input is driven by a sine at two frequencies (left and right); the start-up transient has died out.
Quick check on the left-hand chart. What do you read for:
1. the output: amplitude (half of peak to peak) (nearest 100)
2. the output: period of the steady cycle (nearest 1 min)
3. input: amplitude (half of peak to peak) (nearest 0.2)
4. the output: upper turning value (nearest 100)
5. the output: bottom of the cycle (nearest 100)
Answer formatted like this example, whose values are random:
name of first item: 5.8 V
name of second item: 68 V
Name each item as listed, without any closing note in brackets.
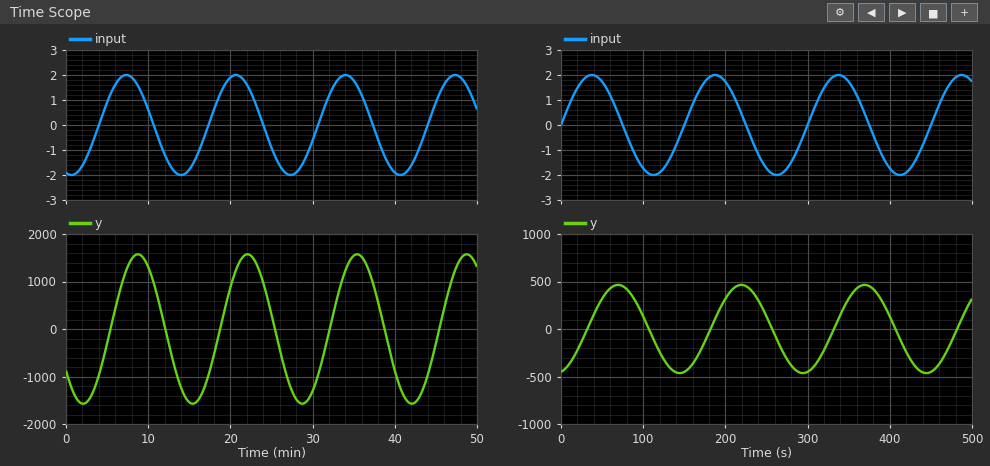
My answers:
the output: amplitude (half of peak to peak): 1600
the output: period of the steady cycle: 13 min
input: amplitude (half of peak to peak): 2.0
the output: upper turning value: 1600
the output: bottom of the cycle: -1600
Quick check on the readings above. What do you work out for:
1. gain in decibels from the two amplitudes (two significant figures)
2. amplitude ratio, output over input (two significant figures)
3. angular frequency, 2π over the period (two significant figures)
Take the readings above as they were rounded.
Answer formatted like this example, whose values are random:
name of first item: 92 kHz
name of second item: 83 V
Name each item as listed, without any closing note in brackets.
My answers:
gain in decibels from the two amplitudes: 58 dB
amplitude ratio, output over input: 800
angular frequency, 2π over the period: 0.48 rad/min
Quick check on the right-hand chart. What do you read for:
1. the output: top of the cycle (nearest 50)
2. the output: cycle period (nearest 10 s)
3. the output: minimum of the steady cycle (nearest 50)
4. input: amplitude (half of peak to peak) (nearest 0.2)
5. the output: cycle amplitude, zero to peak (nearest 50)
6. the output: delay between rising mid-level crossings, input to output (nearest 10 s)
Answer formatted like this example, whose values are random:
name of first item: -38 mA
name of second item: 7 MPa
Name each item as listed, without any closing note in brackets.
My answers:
the output: top of the cycle: 450
the output: cycle period: 150 s
the output: minimum of the steady cycle: -450
input: amplitude (half of peak to peak): 2.0
the output: cycle amplitude, zero to peak: 450
the output: delay between rising mid-level crossings, input to output: 30 s
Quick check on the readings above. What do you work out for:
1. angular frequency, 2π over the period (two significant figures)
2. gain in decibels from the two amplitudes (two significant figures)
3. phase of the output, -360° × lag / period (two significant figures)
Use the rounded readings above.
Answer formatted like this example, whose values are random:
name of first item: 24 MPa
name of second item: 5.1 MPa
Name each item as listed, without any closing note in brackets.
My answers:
angular frequency, 2π over the period: 0.042 rad/s
gain in decibels from the two amplitudes: 47 dB
phase of the output, -360° × lag / period: -72°
